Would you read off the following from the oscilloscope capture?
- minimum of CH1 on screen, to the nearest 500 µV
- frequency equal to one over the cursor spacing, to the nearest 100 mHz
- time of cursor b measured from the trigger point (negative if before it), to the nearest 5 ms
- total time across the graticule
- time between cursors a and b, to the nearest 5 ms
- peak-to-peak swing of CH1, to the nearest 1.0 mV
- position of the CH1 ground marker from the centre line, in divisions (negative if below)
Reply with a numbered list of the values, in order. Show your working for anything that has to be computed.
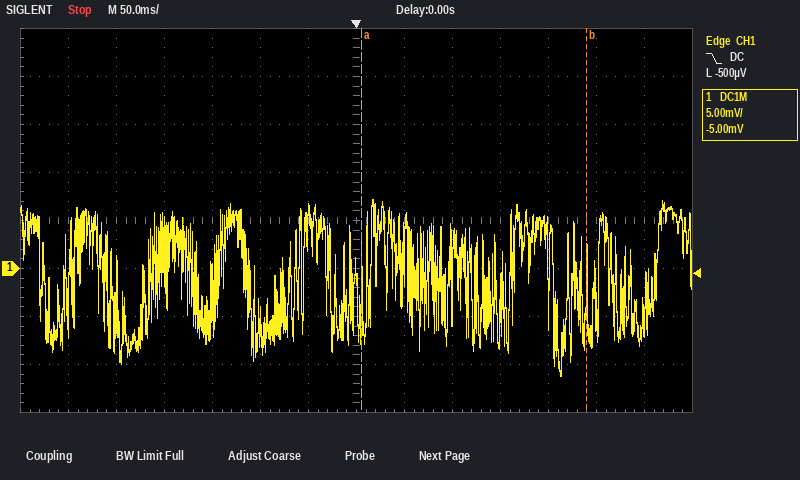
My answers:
1. -11.0 mV
2. 1 / 235 ms ≈ 4.3 Hz
3. +240 ms
4. 700 ms
5. 235 ms
6. 18.0 mV
7. -1.0 div
